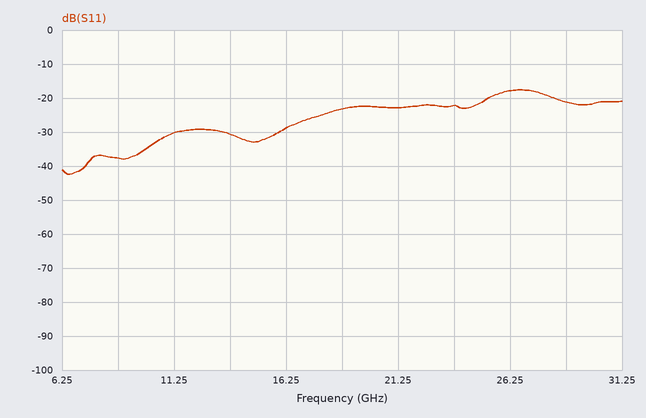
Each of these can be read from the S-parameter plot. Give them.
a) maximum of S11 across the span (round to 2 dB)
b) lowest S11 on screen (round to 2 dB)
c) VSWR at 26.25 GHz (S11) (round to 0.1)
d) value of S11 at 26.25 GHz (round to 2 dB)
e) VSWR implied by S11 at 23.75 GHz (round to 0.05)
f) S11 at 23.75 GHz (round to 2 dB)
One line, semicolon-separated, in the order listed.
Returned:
-18 dB; -42 dB; 1.3; -18 dB; 1.15; -22 dB
